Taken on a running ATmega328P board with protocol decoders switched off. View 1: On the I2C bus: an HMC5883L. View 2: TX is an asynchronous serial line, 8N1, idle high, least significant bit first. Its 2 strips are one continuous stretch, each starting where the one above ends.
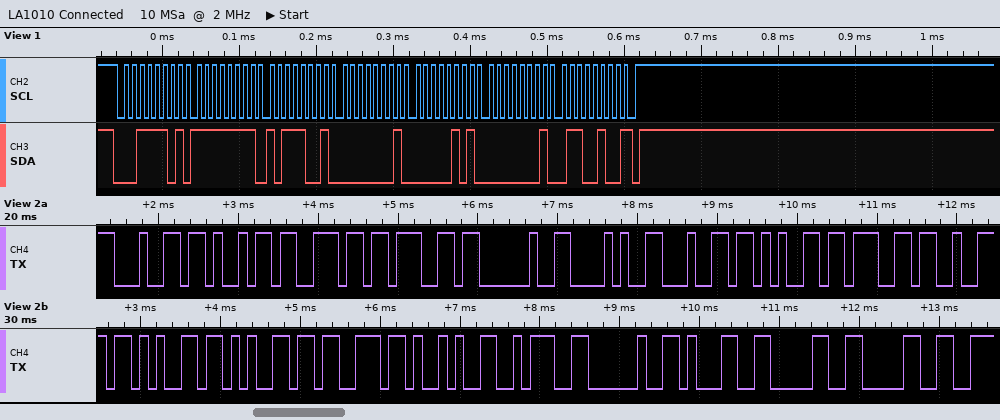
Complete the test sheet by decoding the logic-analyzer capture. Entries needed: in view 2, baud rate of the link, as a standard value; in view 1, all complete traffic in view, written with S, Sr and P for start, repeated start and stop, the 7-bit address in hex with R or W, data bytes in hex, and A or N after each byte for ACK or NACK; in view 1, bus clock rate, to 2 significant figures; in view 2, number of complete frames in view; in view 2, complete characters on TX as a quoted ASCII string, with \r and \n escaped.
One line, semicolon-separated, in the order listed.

9600 baud; S 1ER A FF A B9 A 01 A 05 A 01 A 64 N P; 100 kHz; 19; "ding (degrees): 100"
